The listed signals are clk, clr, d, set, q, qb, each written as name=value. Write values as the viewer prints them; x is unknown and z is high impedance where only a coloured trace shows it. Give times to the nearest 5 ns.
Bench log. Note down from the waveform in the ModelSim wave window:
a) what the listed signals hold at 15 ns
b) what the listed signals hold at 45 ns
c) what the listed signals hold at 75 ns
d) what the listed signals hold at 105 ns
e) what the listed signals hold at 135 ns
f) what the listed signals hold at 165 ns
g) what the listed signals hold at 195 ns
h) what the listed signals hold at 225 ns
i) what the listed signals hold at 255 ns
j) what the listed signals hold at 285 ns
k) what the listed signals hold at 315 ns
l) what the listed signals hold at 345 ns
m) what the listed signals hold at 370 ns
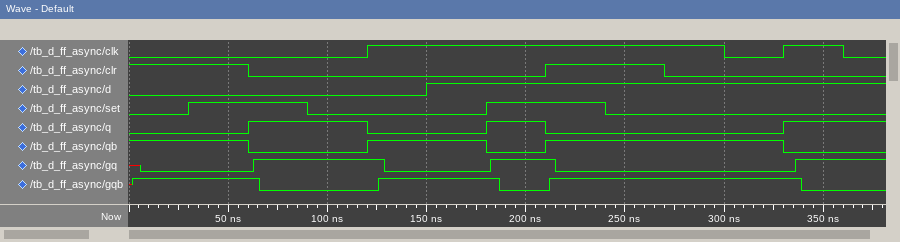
clk=0, clr=1, d=0, set=0, q=0, qb=1
clk=0, clr=1, d=0, set=1, q=0, qb=1
clk=0, clr=0, d=0, set=1, q=1, qb=0
clk=0, clr=0, d=0, set=0, q=1, qb=0
clk=1, clr=0, d=0, set=0, q=0, qb=1
clk=1, clr=0, d=1, set=0, q=0, qb=1
clk=1, clr=0, d=1, set=1, q=1, qb=0
clk=1, clr=1, d=1, set=1, q=0, qb=1
clk=1, clr=1, d=1, set=0, q=0, qb=1
clk=1, clr=0, d=1, set=0, q=0, qb=1
clk=0, clr=0, d=1, set=0, q=0, qb=1
clk=1, clr=0, d=1, set=0, q=1, qb=0
clk=0, clr=0, d=1, set=0, q=1, qb=0
